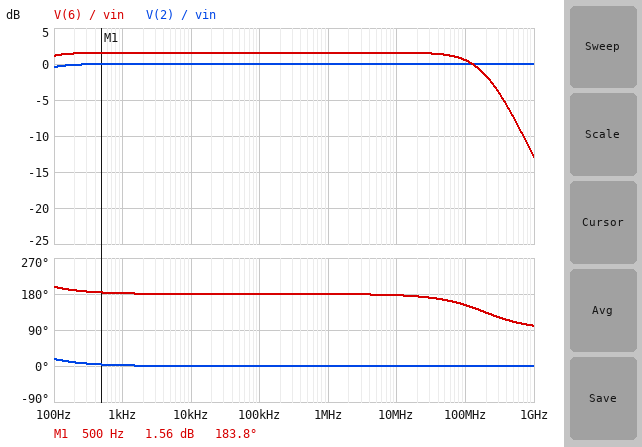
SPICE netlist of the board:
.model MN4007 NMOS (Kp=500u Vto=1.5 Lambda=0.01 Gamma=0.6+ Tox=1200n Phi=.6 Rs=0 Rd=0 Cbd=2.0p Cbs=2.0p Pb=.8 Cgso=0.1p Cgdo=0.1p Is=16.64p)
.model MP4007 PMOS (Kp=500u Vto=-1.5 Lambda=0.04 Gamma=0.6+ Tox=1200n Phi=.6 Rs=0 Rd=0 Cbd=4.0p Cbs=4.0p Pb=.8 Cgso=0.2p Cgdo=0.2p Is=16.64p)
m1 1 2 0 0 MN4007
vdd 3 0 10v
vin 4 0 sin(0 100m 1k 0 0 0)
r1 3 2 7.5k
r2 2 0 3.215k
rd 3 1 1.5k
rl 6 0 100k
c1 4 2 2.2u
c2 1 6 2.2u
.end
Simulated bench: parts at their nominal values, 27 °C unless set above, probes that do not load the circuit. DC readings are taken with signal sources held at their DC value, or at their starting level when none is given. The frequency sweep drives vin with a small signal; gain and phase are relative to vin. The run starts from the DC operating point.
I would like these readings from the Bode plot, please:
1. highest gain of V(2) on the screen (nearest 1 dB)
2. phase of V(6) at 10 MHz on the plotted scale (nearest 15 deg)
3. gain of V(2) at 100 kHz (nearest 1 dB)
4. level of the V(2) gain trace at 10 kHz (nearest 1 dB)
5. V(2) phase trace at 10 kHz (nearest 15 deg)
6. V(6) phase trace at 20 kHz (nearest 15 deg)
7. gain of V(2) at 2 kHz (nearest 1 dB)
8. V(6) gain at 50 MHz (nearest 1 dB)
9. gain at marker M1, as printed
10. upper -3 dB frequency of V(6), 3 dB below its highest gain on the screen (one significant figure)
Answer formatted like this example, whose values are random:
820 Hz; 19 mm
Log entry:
0 dB; 180 deg; 0 dB; 0 dB; 0 deg; 180 deg; 0 dB; 1 dB; 1.56 dB; 200 MHz
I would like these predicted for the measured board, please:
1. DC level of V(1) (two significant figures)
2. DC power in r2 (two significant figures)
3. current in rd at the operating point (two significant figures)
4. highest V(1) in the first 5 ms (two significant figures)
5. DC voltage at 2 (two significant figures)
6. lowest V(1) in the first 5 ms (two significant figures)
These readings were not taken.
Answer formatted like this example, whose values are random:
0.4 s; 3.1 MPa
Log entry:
9.1 V; 2.8 mW; 610 µA; 9.2 V; 3.0 V; 9.0 V
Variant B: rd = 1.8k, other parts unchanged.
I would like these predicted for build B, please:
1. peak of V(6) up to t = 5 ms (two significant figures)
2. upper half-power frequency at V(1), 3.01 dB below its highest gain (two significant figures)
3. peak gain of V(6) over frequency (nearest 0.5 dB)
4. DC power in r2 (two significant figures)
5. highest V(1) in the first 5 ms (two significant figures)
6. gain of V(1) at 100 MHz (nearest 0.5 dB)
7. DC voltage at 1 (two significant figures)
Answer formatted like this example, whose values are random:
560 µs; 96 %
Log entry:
140 mV; 160 MHz; 3.0 dB; 2.8 mW; 9.0 V; 1.5 dB; 8.9 V
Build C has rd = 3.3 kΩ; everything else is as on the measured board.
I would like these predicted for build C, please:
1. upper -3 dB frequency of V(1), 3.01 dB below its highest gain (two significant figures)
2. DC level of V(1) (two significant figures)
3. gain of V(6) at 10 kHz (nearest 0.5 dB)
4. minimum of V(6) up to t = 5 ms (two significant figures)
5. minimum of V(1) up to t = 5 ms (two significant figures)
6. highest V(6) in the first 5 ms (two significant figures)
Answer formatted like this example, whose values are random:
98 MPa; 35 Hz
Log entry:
84 MHz; 8.0 V; 8.0 dB; -260 mV; 7.7 V; 250 mV
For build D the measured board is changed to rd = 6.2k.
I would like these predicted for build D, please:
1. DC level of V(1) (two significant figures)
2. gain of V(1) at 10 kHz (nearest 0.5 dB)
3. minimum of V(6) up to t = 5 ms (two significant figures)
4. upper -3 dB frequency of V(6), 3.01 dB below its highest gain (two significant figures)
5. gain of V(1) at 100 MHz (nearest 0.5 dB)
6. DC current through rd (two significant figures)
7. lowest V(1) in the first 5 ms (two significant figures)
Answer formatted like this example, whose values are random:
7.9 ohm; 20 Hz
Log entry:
6.3 V; 13.0 dB; -460 mV; 42 MHz; 5.0 dB; 600 µA; 5.8 V
